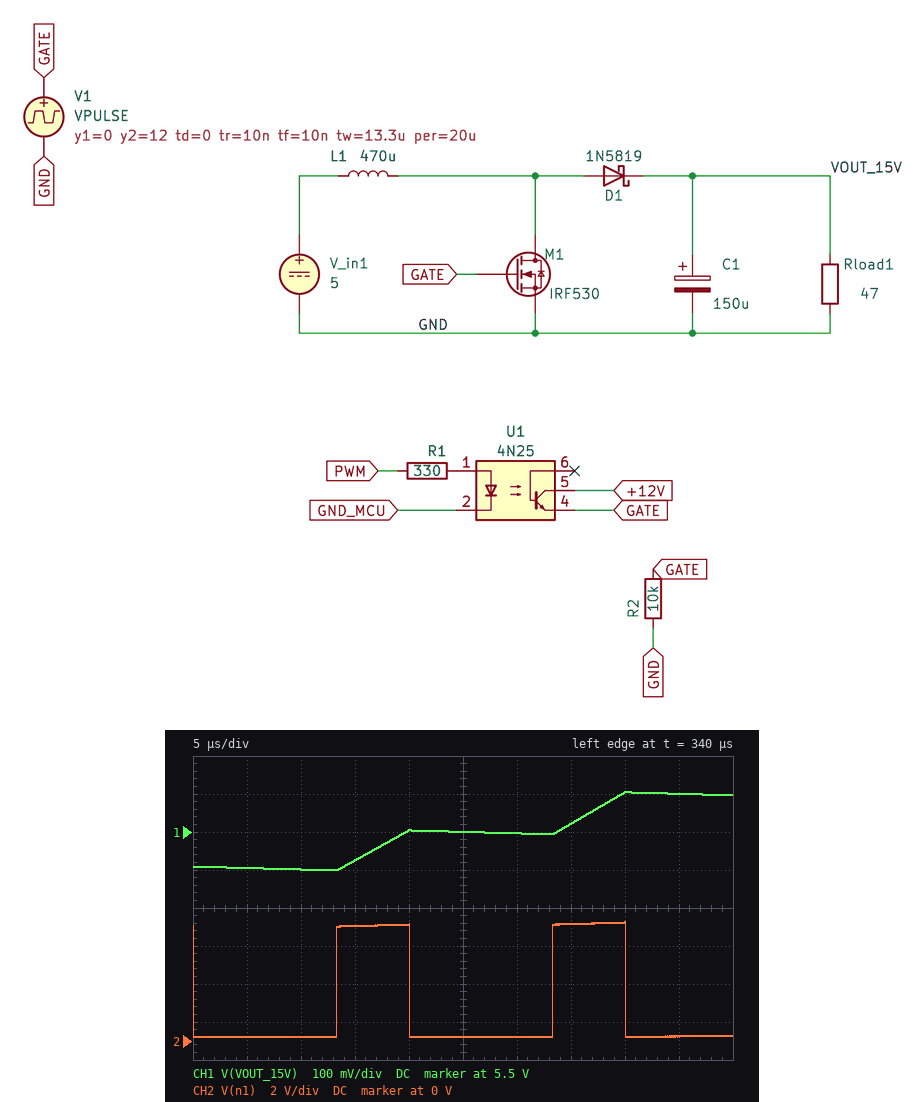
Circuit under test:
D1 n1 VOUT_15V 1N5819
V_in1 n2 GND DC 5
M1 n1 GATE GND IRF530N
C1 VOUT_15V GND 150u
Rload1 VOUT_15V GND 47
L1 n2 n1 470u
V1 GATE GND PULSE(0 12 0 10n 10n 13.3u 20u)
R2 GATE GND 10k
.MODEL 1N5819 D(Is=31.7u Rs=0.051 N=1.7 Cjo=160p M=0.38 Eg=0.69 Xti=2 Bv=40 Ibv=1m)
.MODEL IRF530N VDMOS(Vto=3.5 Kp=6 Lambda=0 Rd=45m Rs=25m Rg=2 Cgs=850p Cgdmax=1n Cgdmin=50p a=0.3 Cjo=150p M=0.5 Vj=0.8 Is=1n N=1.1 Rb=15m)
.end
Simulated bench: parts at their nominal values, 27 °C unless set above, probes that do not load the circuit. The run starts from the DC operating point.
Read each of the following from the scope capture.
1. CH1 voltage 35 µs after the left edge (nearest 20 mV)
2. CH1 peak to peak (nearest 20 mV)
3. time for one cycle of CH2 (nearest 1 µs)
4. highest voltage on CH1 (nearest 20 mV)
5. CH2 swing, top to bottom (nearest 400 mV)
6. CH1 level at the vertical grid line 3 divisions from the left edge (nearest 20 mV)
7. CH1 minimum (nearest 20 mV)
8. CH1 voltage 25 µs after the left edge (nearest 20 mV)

5.52 V
200 mV
20 µs
5.60 V
6.0 V
5.42 V
5.40 V
5.50 V
